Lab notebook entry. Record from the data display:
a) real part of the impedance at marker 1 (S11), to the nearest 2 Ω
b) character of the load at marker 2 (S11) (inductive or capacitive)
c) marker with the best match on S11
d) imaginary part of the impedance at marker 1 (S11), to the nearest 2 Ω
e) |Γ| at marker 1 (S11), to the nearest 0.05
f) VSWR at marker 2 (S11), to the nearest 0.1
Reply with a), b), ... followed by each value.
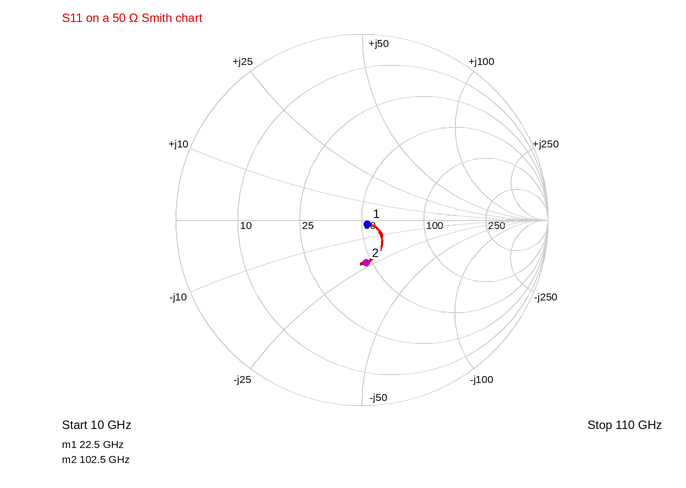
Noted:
a) 52 Ω
b) capacitive
c) marker 1
d) -2 Ω
e) 0.05
f) 1.6
